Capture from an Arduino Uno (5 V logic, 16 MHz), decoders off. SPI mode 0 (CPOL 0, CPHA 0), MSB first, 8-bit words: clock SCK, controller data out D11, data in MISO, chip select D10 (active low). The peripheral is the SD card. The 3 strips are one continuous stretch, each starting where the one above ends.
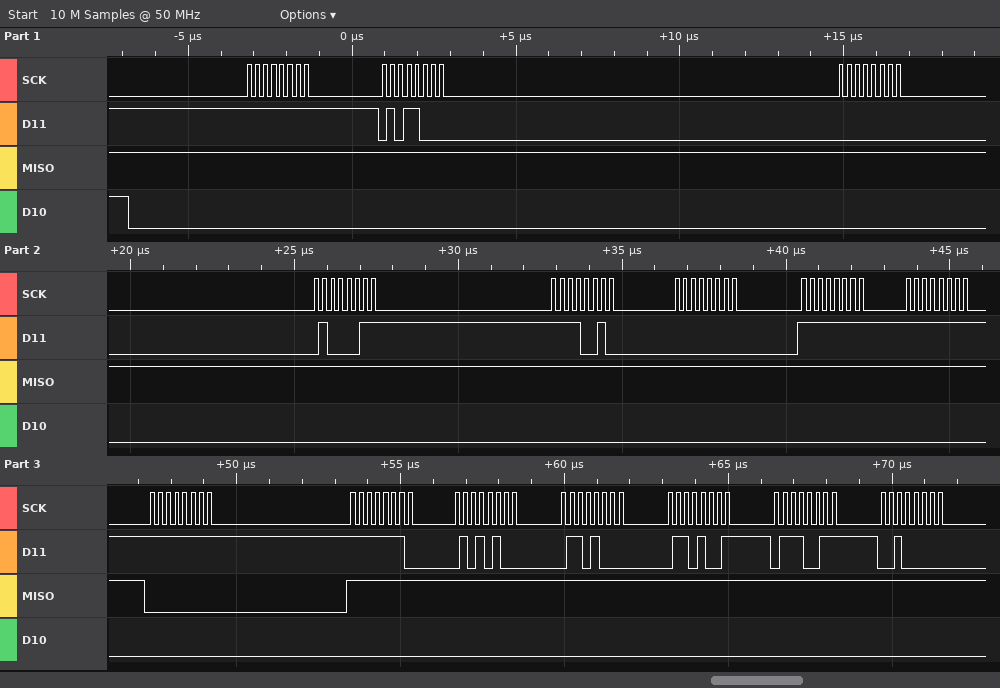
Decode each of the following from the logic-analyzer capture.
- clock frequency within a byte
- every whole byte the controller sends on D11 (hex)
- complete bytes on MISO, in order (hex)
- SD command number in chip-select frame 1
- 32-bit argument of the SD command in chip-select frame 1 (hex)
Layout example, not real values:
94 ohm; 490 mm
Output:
4 MHz; 0xFF 0x58 0x00 0x43 0xF2 0x00 0xFF 0xFF 0xFF 0xFE 0x54 0x68 0x69 0x73 0x20; 0xFF 0xFF 0xFF 0xFF 0xFF 0xFF 0xFF 0xFF 0x00 0xFF 0xFF 0xFF 0xFF 0xFF 0xFF; CMD24; 0x0043F200
